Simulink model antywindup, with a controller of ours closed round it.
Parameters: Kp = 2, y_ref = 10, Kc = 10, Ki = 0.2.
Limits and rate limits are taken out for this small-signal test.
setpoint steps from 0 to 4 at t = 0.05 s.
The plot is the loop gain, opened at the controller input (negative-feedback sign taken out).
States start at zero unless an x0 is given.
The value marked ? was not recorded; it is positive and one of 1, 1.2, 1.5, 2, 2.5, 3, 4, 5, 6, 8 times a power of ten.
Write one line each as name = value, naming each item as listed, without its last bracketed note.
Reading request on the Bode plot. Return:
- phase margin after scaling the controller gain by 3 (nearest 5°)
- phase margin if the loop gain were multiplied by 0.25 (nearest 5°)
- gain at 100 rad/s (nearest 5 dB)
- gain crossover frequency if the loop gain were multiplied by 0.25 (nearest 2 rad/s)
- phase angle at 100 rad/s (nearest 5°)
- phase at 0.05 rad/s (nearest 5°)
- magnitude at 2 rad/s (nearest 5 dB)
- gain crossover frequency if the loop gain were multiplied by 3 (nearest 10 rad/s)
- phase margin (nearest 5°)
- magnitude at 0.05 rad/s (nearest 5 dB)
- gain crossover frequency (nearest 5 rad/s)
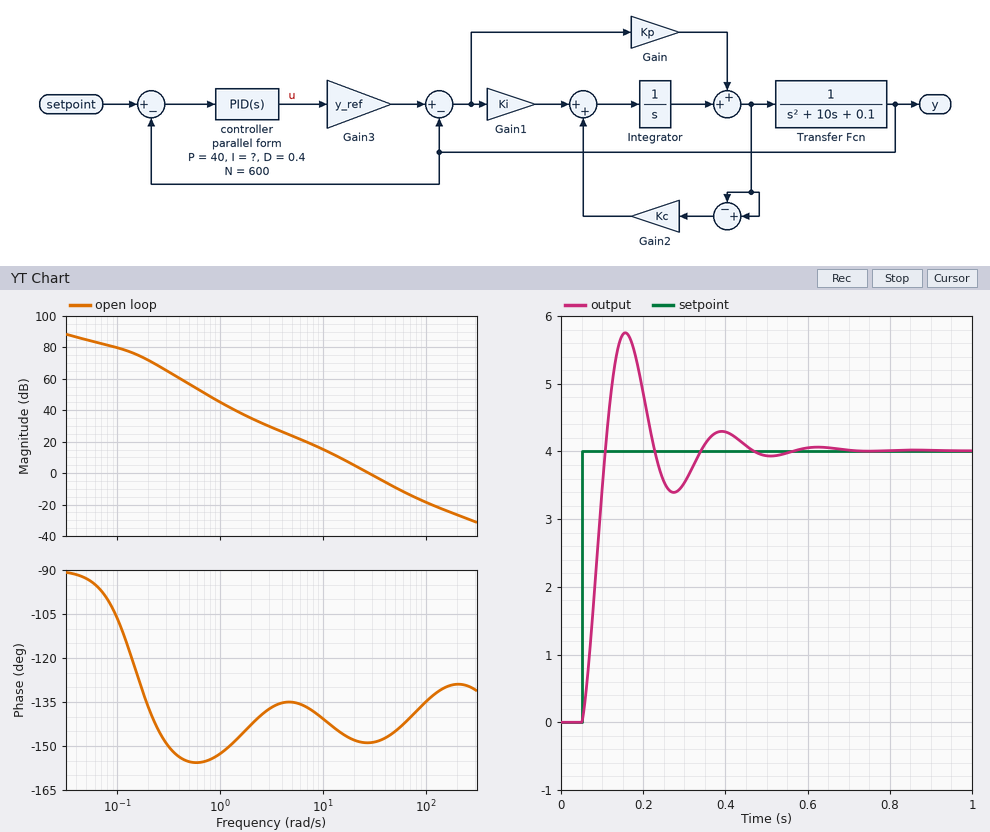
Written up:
phase margin after scaling the controller gain by 3 = 35°
phase margin if the loop gain were multiplied by 0.25 = 35°
gain at 100 rad/s = -20 dB
gain crossover frequency if the loop gain were multiplied by 0.25 = 12 rad/s
phase angle at 100 rad/s = -135°
phase at 0.05 rad/s = -95°
magnitude at 2 rad/s = 35 dB
gain crossover frequency if the loop gain were multiplied by 3 = 50 rad/s
phase margin = 30°
magnitude at 0.05 rad/s = 85 dB
gain crossover frequency = 30 rad/s
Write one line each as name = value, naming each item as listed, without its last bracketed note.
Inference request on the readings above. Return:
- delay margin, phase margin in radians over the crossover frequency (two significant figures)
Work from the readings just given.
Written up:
delay margin, phase margin in radians over the crossover frequency = 0.017 s
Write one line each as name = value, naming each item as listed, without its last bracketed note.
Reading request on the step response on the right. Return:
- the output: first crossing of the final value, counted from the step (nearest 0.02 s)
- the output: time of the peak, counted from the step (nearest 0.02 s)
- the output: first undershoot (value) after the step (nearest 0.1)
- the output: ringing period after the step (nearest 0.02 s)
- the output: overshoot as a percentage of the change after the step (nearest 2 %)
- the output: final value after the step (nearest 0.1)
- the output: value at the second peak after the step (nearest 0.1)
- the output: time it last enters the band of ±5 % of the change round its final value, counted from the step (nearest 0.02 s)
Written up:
the output: first crossing of the final value, counted from the step = 0.06 s
the output: time of the peak, counted from the step = 0.10 s
the output: first undershoot (value) after the step = 3.4
the output: ringing period after the step = 0.24 s
the output: overshoot as a percentage of the change after the step = 44 %
the output: final value after the step = 4.0
the output: value at the second peak after the step = 4.3
the output: time it last enters the band of ±5 % of the change round its final value, counted from the step = 0.38 s
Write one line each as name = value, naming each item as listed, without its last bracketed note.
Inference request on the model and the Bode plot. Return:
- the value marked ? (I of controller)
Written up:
the value marked ? = 80
